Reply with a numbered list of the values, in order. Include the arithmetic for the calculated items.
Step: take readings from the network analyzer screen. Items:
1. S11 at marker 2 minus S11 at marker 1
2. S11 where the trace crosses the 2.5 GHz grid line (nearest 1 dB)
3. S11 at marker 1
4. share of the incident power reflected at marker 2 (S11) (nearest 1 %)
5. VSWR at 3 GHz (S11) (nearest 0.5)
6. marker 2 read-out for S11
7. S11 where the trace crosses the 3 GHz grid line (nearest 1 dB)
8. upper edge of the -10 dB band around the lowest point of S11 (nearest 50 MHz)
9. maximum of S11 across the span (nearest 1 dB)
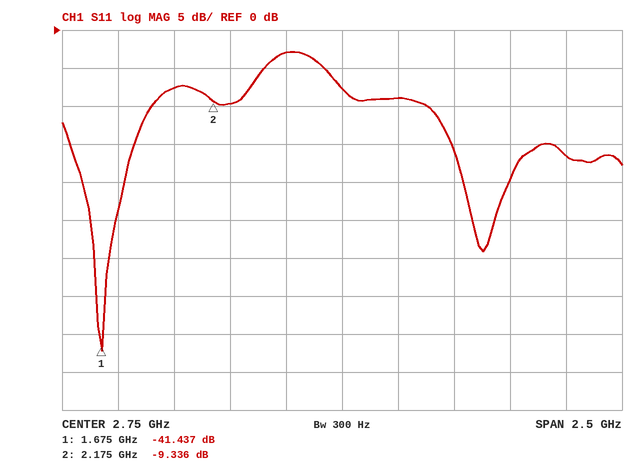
1. -9.336 − (-41.437) = 32.101 dB
2. -3 dB
3. -41.437 dB
4. 10^(-9.336/10) ≈ 12 %
5. |Γ| = 10^(-9/20) = 0.3548; VSWR = (1 + 0.3548)/(1 − 0.3548) ≈ 2.10, so 2.0 to the nearest 0.5
6. -9.336 dB
7. -9 dB
8. 1.90 GHz
9. -3 dB
